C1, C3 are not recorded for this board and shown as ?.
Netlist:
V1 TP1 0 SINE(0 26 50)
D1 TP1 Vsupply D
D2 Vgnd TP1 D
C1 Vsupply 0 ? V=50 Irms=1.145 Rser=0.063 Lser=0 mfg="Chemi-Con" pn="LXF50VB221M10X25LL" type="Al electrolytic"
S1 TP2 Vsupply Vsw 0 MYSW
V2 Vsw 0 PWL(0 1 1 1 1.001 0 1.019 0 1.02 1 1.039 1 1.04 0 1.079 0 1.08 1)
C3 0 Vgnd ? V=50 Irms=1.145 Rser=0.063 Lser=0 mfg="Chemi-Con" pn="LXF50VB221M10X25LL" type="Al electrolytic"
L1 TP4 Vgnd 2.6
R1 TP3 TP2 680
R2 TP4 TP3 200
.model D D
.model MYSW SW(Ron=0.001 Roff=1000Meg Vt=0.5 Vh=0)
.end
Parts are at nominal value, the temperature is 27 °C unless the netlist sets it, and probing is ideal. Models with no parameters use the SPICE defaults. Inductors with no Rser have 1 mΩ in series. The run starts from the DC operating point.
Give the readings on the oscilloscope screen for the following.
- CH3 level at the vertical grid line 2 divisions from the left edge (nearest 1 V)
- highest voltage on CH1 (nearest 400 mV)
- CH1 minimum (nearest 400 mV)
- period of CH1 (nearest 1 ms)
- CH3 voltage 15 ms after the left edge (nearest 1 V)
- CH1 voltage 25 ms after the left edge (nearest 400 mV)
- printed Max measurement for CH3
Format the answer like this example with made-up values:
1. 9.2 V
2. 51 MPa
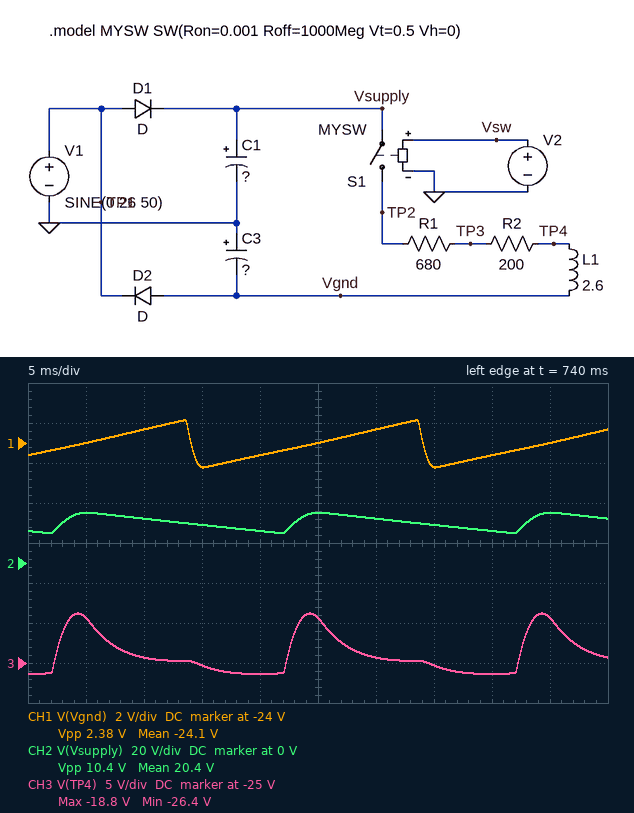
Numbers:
1. -24 V
2. -22.8 V
3. -25.2 V
4. 20 ms
5. -25 V
6. -24.0 V
7. -18.8 V
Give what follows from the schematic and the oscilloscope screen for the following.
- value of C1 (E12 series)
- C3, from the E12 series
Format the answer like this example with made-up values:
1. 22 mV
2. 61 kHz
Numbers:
1. 82 µF
2. 390 µF
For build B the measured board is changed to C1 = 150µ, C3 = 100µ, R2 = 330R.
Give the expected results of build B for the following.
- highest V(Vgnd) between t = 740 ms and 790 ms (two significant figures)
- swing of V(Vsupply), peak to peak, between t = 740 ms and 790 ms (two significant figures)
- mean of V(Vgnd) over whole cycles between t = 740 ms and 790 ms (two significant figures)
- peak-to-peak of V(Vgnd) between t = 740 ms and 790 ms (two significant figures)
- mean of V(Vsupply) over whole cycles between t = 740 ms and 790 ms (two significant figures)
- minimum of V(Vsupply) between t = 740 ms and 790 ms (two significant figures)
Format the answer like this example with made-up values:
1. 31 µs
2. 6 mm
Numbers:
1. -18 V
2. 5.2 V
3. -22 V
4. 7.6 V
5. 23 V
6. 20 V
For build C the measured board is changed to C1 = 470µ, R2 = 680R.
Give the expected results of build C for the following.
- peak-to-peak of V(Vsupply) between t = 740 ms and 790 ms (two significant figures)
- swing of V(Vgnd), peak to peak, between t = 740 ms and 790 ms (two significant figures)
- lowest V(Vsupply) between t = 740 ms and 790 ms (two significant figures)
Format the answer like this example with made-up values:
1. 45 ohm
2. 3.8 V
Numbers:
1. 1.4 V
2. 1.7 V
3. 24 V
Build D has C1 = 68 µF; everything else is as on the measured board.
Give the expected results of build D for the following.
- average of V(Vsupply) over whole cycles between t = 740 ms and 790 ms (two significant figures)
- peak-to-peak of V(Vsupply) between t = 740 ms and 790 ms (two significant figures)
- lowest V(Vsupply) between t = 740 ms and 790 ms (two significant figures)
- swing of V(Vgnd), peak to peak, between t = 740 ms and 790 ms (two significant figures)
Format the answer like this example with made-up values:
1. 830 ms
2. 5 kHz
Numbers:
1. 19 V
2. 12 V
3. 13 V
4. 2.3 V
